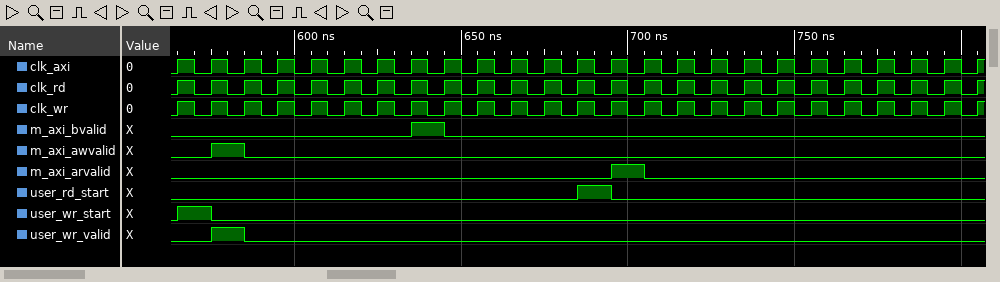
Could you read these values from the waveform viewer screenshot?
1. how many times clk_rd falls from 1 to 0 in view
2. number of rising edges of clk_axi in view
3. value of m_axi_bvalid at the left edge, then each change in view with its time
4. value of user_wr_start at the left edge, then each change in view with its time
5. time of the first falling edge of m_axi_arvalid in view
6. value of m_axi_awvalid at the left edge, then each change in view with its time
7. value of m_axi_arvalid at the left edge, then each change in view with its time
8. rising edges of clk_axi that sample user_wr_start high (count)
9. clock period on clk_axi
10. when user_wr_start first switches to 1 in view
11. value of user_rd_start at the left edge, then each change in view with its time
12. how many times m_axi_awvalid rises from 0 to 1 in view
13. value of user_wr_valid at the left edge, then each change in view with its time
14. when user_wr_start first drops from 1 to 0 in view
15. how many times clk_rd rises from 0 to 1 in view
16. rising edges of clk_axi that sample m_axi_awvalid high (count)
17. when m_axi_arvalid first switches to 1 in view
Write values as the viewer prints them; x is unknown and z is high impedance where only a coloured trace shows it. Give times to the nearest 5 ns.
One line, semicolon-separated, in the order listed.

24; 25; 0, 1 at 635 ns, 0 at 645 ns; 0, 1 at 565 ns, 0 at 575 ns; 705 ns; 0, 1 at 575 ns, 0 at 585 ns; 0, 1 at 695 ns, 0 at 705 ns; 1; 10 ns; 565 ns; 0, 1 at 685 ns, 0 at 695 ns; 1; 0, 1 at 575 ns, 0 at 585 ns; 575 ns; 25; 1; 695 ns
